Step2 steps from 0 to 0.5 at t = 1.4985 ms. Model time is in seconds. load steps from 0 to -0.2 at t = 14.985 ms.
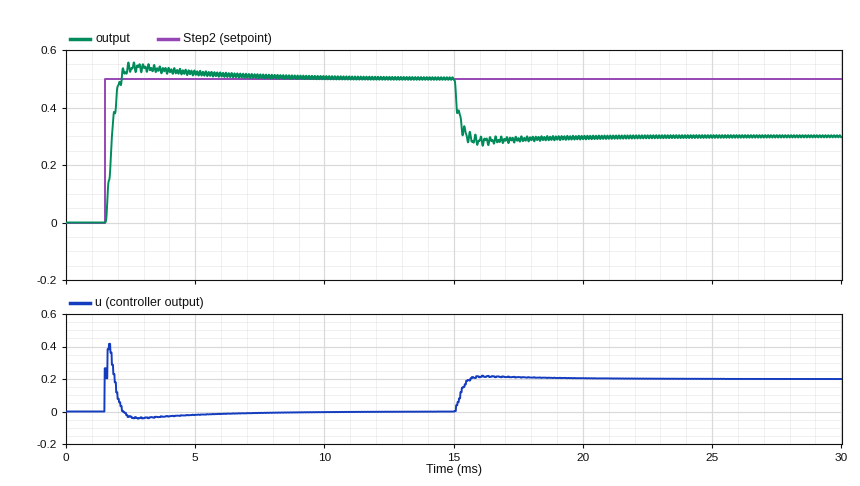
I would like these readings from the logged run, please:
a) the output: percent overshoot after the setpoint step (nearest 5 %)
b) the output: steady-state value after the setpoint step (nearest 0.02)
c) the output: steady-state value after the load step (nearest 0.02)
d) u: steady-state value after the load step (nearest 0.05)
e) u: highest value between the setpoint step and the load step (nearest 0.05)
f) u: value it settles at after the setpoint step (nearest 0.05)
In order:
10 %
0.50
0.30
0.20
0.40
0.00
